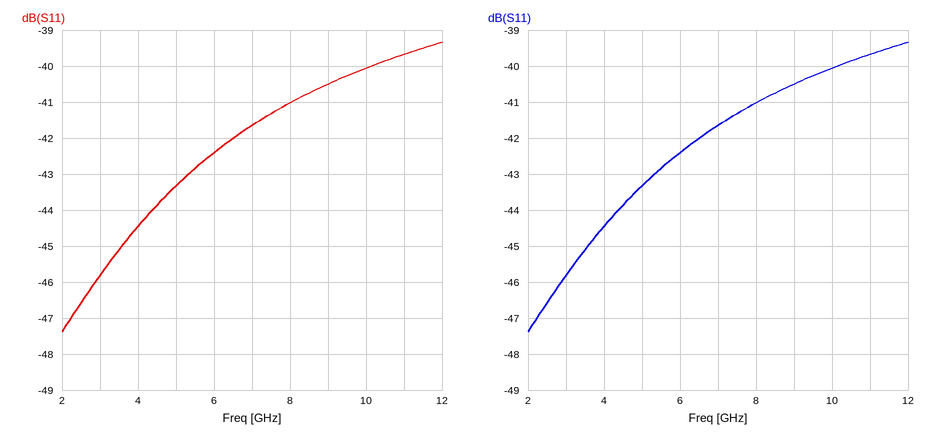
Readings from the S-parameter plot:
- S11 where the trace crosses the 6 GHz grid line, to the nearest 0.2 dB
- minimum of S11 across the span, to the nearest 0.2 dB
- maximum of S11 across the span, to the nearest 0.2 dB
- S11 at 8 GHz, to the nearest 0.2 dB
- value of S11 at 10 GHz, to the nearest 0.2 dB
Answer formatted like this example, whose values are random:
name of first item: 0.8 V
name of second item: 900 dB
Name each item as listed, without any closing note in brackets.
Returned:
S11 where the trace crosses the 6 GHz grid line, to the nearest 0.2 dB: -42.4 dB
minimum of S11 across the span, to the nearest 0.2 dB: -47.4 dB
maximum of S11 across the span, to the nearest 0.2 dB: -39.4 dB
S11 at 8 GHz, to the nearest 0.2 dB: -41.0 dB
value of S11 at 10 GHz, to the nearest 0.2 dB: -40.0 dB
